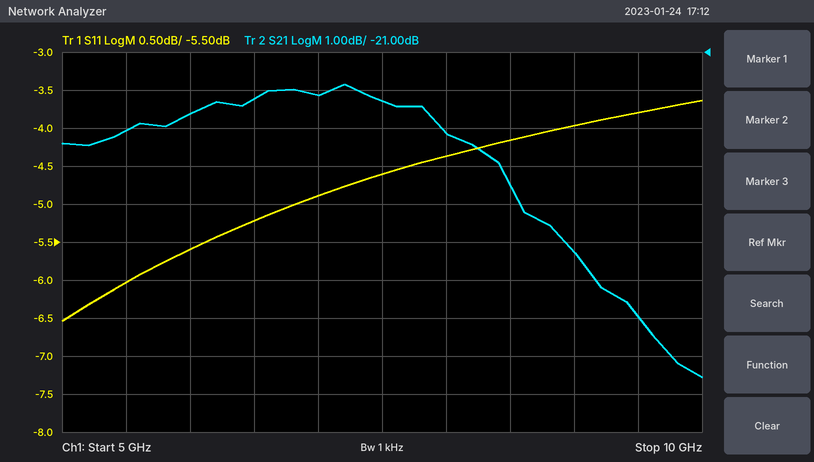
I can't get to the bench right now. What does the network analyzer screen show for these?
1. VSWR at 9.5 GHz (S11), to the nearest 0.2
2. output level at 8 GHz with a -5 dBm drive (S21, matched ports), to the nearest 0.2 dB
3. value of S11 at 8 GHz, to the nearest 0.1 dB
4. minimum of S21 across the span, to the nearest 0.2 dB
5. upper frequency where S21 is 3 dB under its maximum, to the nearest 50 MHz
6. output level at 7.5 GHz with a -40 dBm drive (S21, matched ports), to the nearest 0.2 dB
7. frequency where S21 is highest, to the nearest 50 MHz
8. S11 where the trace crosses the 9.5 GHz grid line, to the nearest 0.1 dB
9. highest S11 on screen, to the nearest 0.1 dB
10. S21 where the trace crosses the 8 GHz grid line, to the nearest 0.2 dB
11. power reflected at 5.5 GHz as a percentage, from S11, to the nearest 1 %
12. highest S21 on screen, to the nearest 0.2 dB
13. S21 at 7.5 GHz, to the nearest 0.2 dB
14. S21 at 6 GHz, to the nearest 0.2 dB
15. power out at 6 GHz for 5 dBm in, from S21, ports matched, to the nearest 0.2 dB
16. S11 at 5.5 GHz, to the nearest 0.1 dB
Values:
4.6
-28.2 dBm
-4.4 dB
-29.6 dB
8.55 GHz
-62.2 dBm
7.20 GHz
-3.8 dB
-3.6 dB
-23.2 dB
25 %
-21.8 dB
-22.2 dB
-22.6 dB
-17.6 dBm
-6.0 dB
